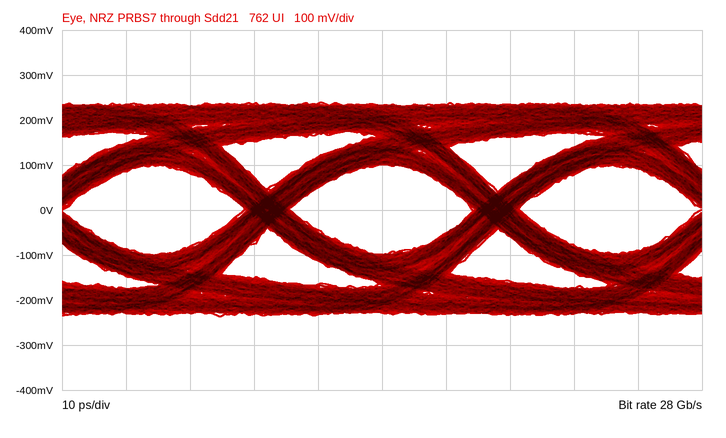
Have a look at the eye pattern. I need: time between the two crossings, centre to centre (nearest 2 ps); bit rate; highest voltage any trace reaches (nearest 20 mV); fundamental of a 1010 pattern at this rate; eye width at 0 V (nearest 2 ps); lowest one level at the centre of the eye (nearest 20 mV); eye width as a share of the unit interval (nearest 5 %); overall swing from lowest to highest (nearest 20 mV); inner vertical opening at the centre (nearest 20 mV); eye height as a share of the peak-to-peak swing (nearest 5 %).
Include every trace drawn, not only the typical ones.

36 ps
28 Gb/s
240 mV
14 GHz
28 ps
100 mV
80 %
480 mV
200 mV
40 %
